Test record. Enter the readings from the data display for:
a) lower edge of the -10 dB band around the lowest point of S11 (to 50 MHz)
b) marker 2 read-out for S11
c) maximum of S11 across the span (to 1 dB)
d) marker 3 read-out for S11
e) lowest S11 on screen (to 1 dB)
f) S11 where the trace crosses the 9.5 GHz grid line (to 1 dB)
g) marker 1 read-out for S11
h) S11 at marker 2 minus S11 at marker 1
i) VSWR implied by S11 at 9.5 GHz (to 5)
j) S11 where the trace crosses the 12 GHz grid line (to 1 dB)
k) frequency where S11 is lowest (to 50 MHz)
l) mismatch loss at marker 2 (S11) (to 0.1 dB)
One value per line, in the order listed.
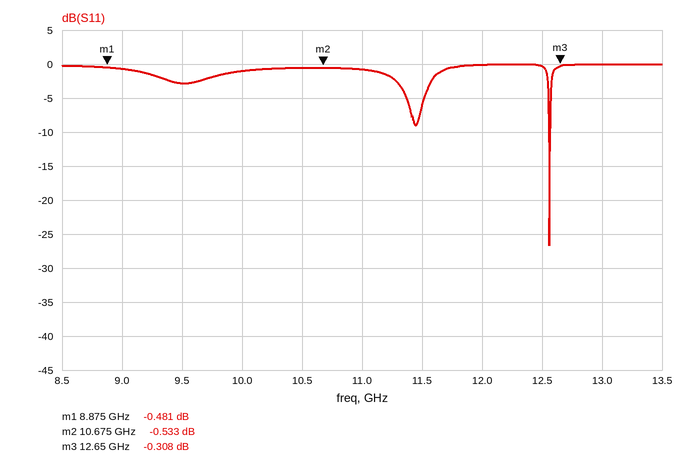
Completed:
12.55 GHz
-0.533 dB
0 dB
-0.308 dB
-27 dB
-3 dB
-0.481 dB
-0.052 dB
5
0 dB
12.55 GHz
9.4 dB
